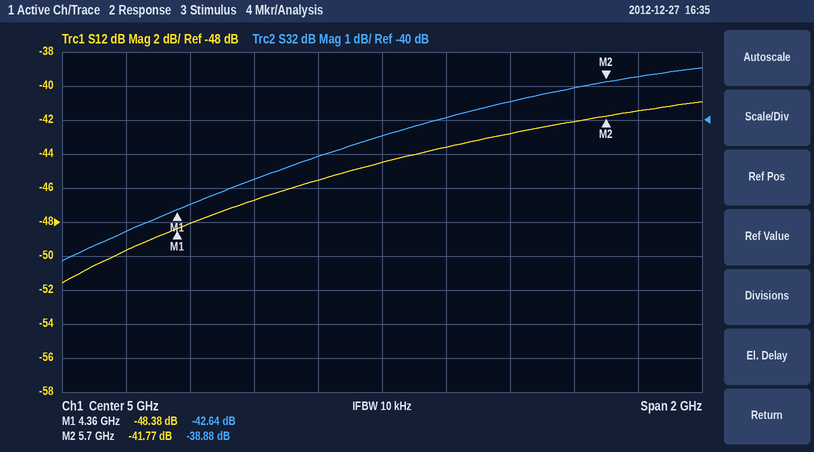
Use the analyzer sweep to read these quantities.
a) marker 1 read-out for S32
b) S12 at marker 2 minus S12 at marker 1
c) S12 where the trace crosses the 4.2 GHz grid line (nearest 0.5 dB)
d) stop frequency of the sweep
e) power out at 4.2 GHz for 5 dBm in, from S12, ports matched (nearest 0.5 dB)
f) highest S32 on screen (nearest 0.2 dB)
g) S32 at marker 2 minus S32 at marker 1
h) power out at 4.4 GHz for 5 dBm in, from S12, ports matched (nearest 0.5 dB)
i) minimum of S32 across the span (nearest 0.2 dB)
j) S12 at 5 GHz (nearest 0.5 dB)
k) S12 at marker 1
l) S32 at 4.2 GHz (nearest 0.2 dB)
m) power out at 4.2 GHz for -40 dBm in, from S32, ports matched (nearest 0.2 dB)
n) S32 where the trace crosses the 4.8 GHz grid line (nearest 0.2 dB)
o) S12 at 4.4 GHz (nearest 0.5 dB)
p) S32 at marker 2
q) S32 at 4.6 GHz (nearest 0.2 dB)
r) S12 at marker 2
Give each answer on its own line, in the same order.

-42.64 dB
6.61 dB
-49.5 dB
6 GHz
-44.5 dBm
-38.4 dB
3.76 dB
-43.0 dBm
-44.2 dB
-44.5 dB
-48.38 dB
-43.2 dB
-83.2 dBm
-41.0 dB
-48.0 dB
-38.88 dB
-41.8 dB
-41.77 dB
